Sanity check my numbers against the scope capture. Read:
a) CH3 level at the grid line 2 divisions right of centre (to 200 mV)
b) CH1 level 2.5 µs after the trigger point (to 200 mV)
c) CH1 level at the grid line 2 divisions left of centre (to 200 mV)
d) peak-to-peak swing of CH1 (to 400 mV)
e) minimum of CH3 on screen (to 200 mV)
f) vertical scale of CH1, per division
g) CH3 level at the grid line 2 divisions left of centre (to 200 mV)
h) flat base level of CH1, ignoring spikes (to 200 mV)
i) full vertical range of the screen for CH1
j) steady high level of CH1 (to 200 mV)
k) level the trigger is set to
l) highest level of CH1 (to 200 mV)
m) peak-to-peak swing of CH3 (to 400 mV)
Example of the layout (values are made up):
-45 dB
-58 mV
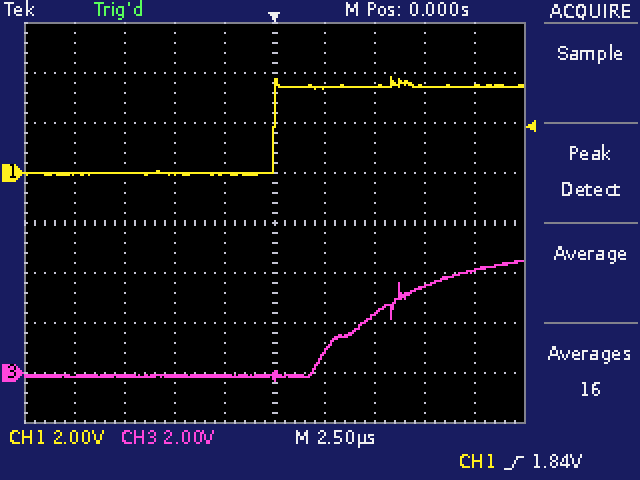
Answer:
2.4 V
3.4 V
0.0 V
4.0 V
-400 mV
2 V
-200 mV
0.0 V
16 V
3.4 V
1.84 V
3.8 V
4.8 V
